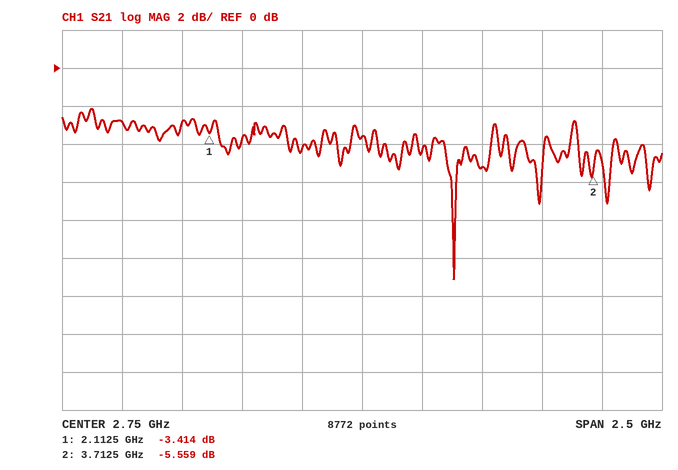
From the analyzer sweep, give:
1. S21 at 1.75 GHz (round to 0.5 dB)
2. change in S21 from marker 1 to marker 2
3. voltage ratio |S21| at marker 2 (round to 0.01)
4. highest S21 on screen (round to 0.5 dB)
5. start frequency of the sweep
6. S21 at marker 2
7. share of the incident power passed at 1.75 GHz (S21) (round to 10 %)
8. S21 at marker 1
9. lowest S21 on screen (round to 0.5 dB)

-3.0 dB
-2.145 dB
0.53
-2.0 dB
1.5 GHz
-5.559 dB
50 %
-3.414 dB
-11.0 dB
